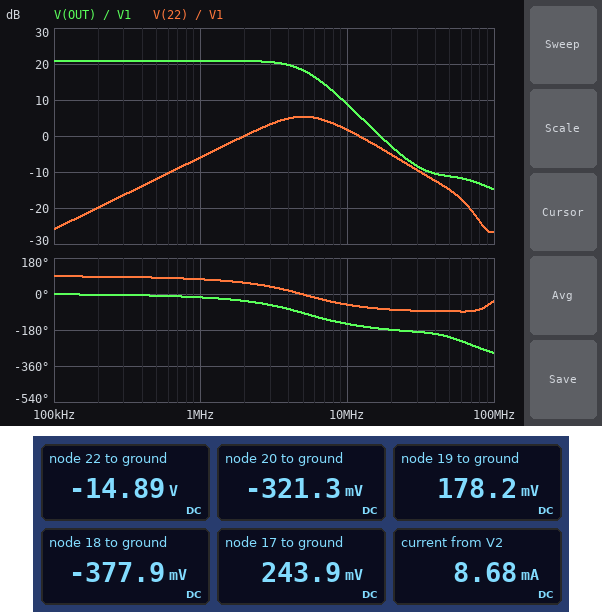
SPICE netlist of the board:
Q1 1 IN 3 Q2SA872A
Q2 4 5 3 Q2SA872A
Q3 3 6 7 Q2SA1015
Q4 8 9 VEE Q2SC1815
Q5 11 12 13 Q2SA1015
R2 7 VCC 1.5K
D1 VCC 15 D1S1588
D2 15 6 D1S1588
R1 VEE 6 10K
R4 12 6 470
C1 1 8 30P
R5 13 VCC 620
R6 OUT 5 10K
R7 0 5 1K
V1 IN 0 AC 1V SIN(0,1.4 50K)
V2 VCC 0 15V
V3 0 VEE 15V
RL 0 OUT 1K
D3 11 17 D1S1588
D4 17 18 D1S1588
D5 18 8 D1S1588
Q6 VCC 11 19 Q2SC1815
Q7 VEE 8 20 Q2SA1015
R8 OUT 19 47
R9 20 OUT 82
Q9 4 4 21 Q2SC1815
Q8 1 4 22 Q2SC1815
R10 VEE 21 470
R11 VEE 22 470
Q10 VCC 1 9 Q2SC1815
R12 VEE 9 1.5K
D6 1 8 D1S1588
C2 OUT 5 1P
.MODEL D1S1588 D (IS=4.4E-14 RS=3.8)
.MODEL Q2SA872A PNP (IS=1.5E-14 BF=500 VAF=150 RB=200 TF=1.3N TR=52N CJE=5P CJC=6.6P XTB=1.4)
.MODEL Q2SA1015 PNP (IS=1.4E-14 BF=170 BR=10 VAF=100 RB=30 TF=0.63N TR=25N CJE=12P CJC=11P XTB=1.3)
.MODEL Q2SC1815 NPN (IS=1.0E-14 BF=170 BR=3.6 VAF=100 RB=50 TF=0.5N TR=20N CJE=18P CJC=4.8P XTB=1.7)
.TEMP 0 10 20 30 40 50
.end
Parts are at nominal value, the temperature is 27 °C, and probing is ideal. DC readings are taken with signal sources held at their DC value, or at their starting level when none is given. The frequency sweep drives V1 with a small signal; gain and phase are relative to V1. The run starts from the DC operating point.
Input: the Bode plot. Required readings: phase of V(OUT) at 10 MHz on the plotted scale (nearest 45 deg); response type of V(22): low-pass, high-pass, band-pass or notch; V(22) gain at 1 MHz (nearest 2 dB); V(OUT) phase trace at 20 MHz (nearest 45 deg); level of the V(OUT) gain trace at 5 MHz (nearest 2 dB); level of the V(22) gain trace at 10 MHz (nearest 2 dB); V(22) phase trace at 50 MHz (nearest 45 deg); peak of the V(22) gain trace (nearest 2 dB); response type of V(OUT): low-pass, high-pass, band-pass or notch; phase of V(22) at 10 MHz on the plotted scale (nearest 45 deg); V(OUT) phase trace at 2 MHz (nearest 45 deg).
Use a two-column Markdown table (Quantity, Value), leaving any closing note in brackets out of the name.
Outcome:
| Quantity | Value |
|---|---|
| phase of V(OUT) at 10 MHz on the plotted scale | -135 deg |
| response type of V(22): low-pass, high-pass, band-pass or notch | band-pass |
| V(22) gain at 1 MHz | -6 dB |
| V(OUT) phase trace at 20 MHz | -180 deg |
| level of the V(OUT) gain trace at 5 MHz | 18 dB |
| level of the V(22) gain trace at 10 MHz | 2 dB |
| V(22) phase trace at 50 MHz | -90 deg |
| peak of the V(22) gain trace | 6 dB |
| response type of V(OUT): low-pass, high-pass, band-pass or notch | low-pass |
| phase of V(22) at 10 MHz on the plotted scale | -45 deg |
| V(OUT) phase trace at 2 MHz | -45 deg |
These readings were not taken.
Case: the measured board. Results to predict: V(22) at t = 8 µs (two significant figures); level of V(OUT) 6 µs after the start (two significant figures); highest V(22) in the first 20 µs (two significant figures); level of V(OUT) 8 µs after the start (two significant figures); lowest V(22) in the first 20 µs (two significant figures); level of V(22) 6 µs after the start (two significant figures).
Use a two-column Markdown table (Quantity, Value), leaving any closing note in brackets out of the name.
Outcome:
| Quantity | Value |
|---|---|
| V(22) at t = 8 µs | -15 V |
| level of V(OUT) 6 µs after the start | 13 V |
| highest V(22) in the first 20 µs | -15 V |
| level of V(OUT) 8 µs after the start | 9.2 V |
| lowest V(22) in the first 20 µs | -15 V |
| level of V(22) 6 µs after the start | -15 V |
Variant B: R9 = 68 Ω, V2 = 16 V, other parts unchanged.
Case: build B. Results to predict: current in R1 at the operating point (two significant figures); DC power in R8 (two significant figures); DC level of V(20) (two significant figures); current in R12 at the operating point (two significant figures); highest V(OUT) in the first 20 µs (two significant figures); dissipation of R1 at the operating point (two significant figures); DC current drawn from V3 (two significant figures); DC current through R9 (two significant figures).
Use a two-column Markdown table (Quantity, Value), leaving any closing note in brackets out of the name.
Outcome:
| Quantity | Value |
|---|---|
| current in R1 at the operating point | 3.0 mA |
| DC power in R8 | 870 µW |
| DC level of V(20) | -300 mV |
| current in R12 at the operating point | 440 µA |
| highest V(OUT) in the first 20 µs | 14 V |
| dissipation of R1 at the operating point | 88 mW |
| DC current drawn from V3 | 9.2 mA |
| DC current through R9 | 4.3 mA |
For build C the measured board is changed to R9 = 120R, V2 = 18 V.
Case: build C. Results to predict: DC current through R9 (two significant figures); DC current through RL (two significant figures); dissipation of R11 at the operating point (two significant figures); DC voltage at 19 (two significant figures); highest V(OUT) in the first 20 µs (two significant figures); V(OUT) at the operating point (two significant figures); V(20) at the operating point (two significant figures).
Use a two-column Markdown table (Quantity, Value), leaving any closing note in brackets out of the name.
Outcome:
| Quantity | Value |
|---|---|
| DC current through R9 | 3.1 mA |
| DC current through RL | 3.8 µA |
| dissipation of R11 at the operating point | 25 µW |
| DC voltage at 19 | 140 mV |
| highest V(OUT) in the first 20 µs | 15 V |
| V(OUT) at the operating point | -3.8 mV |
| V(20) at the operating point | -370 mV |
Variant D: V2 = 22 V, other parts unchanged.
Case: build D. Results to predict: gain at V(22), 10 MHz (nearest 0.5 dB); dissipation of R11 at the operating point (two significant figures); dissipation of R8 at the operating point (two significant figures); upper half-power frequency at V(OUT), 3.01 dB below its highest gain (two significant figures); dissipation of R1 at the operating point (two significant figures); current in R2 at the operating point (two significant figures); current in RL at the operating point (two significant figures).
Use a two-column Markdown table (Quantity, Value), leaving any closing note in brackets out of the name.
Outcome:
| Quantity | Value |
|---|---|
| gain at V(22), 10 MHz | 2.0 dB |
| dissipation of R11 at the operating point | 25 µW |
| dissipation of R8 at the operating point | 710 µW |
| upper half-power frequency at V(OUT), 3.01 dB below its highest gain | 5.3 MHz |
| dissipation of R1 at the operating point | 130 mW |
| current in R2 at the operating point | 470 µA |
| current in RL at the operating point | 4.0 µA |
